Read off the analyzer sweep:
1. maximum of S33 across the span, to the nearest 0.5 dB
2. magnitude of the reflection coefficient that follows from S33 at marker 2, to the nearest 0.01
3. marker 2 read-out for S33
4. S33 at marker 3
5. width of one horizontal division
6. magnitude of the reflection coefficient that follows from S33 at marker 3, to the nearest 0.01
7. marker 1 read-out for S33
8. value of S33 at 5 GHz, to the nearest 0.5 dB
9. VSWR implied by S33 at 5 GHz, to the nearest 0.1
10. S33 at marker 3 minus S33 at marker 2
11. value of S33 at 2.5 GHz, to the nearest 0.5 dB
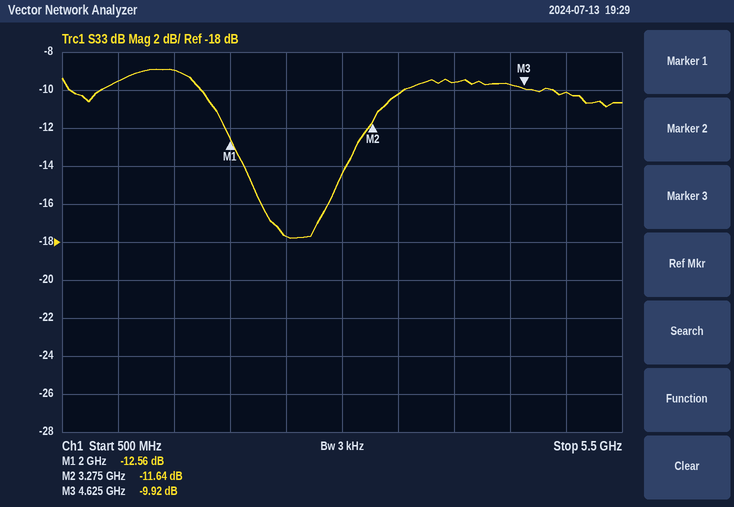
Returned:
-9.0 dB
0.26
-11.64 dB
-9.92 dB
500 MHz
0.32
-12.56 dB
-10.0 dB
1.9
1.72 dB
-17.5 dB
